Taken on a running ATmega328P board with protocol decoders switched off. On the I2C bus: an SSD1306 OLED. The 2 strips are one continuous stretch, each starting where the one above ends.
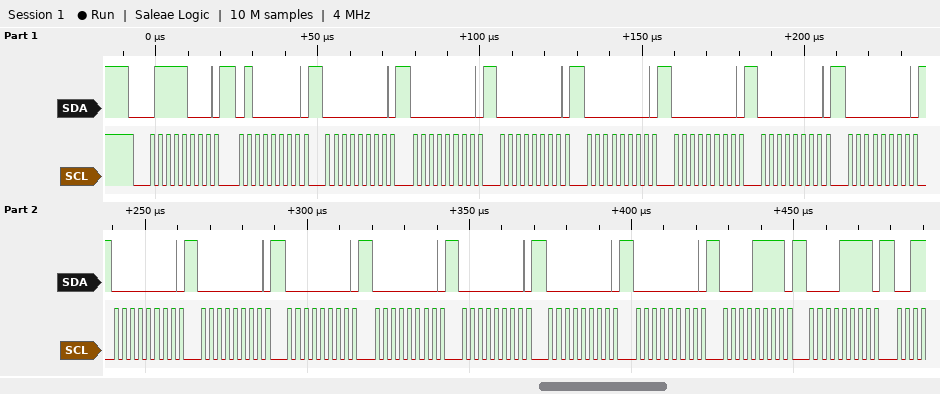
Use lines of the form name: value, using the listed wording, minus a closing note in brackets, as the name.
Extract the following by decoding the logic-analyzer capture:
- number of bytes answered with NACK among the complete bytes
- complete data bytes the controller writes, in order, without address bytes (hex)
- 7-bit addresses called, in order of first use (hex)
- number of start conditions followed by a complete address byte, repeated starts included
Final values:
number of bytes answered with NACK among the complete bytes: 0
complete data bytes the controller writes, in order, without address bytes: 40 00 00 00 00 00 00 00 00 00 00 00 00 00 00 0F 0F
7-bit addresses called, in order of first use: 0x3C
number of start conditions followed by a complete address byte, repeated starts included: 1
